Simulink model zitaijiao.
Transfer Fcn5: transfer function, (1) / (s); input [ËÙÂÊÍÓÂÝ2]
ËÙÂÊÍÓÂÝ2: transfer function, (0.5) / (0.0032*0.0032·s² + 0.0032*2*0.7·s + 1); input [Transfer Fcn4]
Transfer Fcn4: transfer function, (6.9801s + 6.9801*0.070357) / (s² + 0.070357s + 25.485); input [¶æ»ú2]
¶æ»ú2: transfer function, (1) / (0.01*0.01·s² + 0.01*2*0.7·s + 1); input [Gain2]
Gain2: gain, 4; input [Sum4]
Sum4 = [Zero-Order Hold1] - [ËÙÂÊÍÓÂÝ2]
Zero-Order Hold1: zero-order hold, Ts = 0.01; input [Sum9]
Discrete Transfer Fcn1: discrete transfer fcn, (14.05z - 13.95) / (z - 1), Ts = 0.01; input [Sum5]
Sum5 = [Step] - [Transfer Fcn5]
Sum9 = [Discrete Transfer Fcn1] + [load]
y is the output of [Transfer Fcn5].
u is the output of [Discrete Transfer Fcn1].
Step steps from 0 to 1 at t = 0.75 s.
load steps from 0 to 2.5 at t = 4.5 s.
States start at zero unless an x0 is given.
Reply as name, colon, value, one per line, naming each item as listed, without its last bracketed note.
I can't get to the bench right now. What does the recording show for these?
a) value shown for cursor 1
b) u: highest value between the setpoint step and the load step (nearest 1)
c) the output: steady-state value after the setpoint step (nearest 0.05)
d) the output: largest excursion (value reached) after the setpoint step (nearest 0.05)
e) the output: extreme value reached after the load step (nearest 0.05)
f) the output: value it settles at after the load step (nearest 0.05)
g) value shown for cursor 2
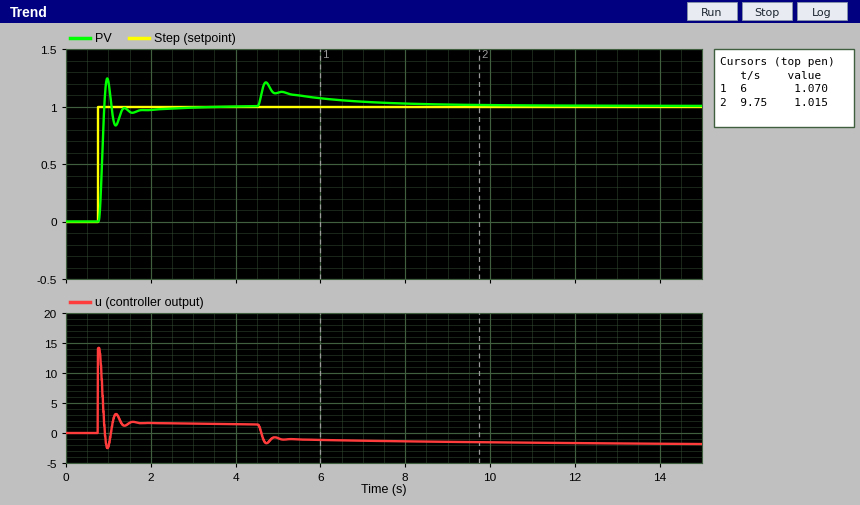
value shown for cursor 1: 1.070
u: highest value between the setpoint step and the load step: 14
the output: steady-state value after the setpoint step: 1.00
the output: largest excursion (value reached) after the setpoint step: 1.25
the output: extreme value reached after the load step: 1.20
the output: value it settles at after the load step: 1.00
value shown for cursor 2: 1.015
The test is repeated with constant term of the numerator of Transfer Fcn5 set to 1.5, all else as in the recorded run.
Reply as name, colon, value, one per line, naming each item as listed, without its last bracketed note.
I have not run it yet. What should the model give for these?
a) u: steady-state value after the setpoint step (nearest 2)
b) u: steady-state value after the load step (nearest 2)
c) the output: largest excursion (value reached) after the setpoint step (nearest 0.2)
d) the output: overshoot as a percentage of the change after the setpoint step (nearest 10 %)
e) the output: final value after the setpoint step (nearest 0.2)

u: steady-state value after the setpoint step: 0
u: steady-state value after the load step: -2
the output: largest excursion (value reached) after the setpoint step: 1.4
the output: overshoot as a percentage of the change after the setpoint step: 50 %
the output: final value after the setpoint step: 1.0
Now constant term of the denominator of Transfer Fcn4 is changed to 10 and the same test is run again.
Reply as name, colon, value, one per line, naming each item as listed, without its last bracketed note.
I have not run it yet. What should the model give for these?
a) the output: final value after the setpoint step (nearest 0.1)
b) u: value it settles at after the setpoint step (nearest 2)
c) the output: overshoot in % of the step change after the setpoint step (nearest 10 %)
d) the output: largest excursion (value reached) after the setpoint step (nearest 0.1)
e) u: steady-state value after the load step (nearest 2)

the output: final value after the setpoint step: 1.0
u: value it settles at after the setpoint step: 0
the output: overshoot in % of the step change after the setpoint step: 30 %
the output: largest excursion (value reached) after the setpoint step: 1.3
u: steady-state value after the load step: -2
